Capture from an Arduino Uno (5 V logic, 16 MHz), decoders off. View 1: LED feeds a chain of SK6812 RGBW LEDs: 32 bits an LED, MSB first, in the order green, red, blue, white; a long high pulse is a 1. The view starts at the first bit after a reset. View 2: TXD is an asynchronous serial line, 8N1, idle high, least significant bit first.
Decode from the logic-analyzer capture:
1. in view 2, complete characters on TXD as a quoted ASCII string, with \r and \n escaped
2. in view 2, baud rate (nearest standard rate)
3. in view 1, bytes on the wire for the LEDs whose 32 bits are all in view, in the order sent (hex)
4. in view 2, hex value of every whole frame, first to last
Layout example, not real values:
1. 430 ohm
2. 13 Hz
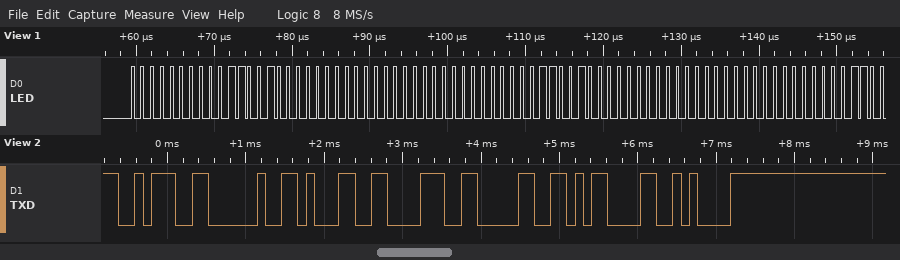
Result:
1. ": 180\r\n"
2. 9600 baud
3. 00 32 00 00 00 32 00 00
4. 3A 20 31 38 30 0D 0A
